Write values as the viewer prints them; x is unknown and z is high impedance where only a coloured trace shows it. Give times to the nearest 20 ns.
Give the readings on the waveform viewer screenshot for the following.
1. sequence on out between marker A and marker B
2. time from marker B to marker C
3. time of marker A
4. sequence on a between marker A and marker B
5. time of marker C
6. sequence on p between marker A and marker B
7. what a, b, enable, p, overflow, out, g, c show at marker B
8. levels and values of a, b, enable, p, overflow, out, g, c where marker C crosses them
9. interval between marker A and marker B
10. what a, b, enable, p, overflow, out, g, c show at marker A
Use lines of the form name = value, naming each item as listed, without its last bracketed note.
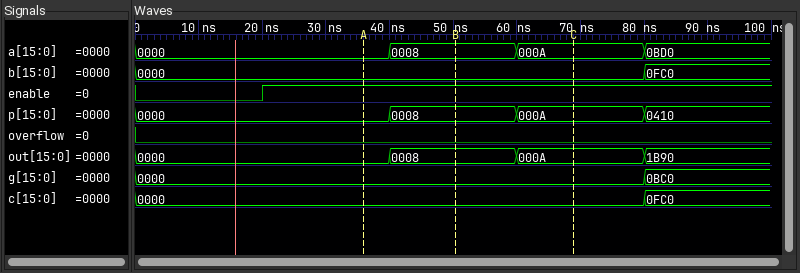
sequence on out between marker A and marker B = 0000, 0008
time from marker B to marker C = 20 ns
time of marker A = 40 ns
sequence on a between marker A and marker B = 0000, 0008
time of marker C = 60 ns
sequence on p between marker A and marker B = 0000, 0008
what a, b, enable, p, overflow, out, g, c show at marker B = a=0008, b=0000, enable=1, p=0008, overflow=0, out=0008, g=0000, c=0000
levels and values of a, b, enable, p, overflow, out, g, c where marker C crosses them = a=000A, b=0000, enable=1, p=000A, overflow=0, out=000A, g=0000, c=0000
interval between marker A and marker B = 20 ns
what a, b, enable, p, overflow, out, g, c show at marker A = a=0000, b=0000, enable=1, p=0000, overflow=0, out=0000, g=0000, c=0000
